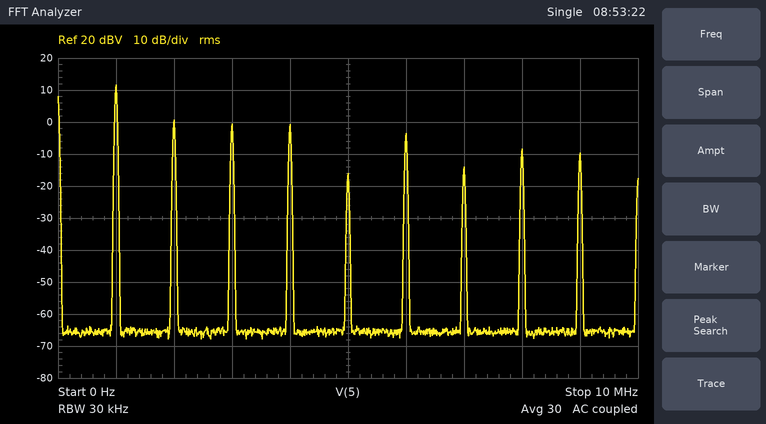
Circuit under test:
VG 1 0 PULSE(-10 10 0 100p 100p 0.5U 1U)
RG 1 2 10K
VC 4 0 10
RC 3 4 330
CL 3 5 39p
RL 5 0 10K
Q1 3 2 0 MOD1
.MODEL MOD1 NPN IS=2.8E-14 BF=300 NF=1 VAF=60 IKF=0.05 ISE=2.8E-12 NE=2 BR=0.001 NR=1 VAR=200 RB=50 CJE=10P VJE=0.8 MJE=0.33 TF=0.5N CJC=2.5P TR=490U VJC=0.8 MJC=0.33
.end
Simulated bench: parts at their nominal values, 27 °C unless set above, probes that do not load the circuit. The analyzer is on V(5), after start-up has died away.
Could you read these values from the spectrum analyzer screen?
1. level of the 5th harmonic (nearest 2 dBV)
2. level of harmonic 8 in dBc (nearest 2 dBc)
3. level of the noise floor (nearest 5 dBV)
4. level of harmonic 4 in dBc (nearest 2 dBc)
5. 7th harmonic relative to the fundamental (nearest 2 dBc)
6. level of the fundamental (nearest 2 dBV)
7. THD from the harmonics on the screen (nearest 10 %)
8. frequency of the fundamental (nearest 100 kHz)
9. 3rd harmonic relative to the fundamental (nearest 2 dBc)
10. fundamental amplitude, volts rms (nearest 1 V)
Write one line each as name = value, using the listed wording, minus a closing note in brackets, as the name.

level of the 5th harmonic = -16 dBV
level of harmonic 8 in dBc = -20 dBc
level of the noise floor = -65 dBV
level of harmonic 4 in dBc = -12 dBc
7th harmonic relative to the fundamental = -26 dBc
level of the fundamental = 12 dBV
THD from the harmonics on the screen = 50 %
frequency of the fundamental = 1.0 MHz
3rd harmonic relative to the fundamental = -12 dBc
fundamental amplitude, volts rms = 4 V
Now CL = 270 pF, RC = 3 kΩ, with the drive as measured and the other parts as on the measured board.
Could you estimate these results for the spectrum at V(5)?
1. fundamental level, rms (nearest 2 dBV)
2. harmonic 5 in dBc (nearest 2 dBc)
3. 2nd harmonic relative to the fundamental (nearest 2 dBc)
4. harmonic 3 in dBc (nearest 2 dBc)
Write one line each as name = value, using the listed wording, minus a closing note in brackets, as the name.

fundamental level, rms = 10 dBV
harmonic 5 in dBc = -18 dBc
2nd harmonic relative to the fundamental = -8 dBc
harmonic 3 in dBc = -20 dBc
